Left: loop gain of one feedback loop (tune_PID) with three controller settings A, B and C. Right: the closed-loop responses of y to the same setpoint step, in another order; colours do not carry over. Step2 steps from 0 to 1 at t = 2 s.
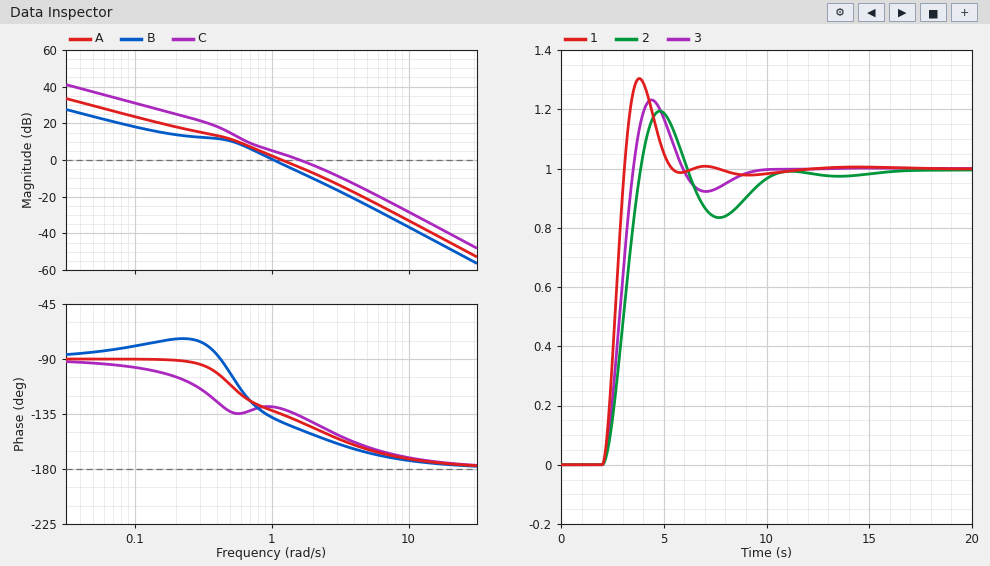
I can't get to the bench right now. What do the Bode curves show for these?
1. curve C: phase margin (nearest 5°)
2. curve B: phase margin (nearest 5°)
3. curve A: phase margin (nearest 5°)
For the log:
45°
40°
45°
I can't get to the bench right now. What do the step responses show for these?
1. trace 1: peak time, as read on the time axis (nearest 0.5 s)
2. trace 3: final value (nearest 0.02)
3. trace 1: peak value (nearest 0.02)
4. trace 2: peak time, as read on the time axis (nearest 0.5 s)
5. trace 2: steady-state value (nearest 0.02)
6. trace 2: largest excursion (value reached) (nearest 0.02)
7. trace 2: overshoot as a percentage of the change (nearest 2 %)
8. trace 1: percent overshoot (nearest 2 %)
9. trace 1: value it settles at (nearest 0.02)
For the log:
4.0 s
1.00
1.30
5.0 s
1.00
1.20
20 %
30 %
1.00
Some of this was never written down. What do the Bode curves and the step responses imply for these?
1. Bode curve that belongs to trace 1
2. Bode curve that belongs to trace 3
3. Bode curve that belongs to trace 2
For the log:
C
A
B
